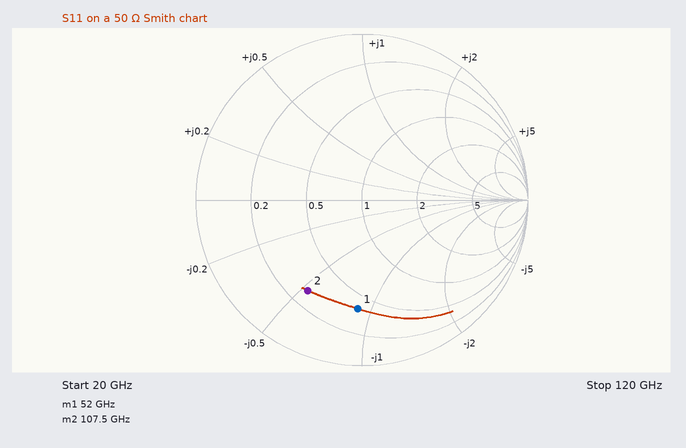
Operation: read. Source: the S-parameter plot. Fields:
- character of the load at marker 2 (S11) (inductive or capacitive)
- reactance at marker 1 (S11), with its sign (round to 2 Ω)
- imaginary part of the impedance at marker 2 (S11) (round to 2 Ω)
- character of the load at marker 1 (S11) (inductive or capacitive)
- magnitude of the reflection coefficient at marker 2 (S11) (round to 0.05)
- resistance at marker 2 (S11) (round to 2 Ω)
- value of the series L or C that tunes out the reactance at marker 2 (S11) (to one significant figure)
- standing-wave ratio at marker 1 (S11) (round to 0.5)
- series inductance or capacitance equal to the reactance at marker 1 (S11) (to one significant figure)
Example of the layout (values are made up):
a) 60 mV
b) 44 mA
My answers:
a) capacitive
b) -44 Ω
c) -26 Ω
d) capacitive
e) 0.65
f) 14 Ω
g) 40 pH
h) 5.0
i) 70 fF
